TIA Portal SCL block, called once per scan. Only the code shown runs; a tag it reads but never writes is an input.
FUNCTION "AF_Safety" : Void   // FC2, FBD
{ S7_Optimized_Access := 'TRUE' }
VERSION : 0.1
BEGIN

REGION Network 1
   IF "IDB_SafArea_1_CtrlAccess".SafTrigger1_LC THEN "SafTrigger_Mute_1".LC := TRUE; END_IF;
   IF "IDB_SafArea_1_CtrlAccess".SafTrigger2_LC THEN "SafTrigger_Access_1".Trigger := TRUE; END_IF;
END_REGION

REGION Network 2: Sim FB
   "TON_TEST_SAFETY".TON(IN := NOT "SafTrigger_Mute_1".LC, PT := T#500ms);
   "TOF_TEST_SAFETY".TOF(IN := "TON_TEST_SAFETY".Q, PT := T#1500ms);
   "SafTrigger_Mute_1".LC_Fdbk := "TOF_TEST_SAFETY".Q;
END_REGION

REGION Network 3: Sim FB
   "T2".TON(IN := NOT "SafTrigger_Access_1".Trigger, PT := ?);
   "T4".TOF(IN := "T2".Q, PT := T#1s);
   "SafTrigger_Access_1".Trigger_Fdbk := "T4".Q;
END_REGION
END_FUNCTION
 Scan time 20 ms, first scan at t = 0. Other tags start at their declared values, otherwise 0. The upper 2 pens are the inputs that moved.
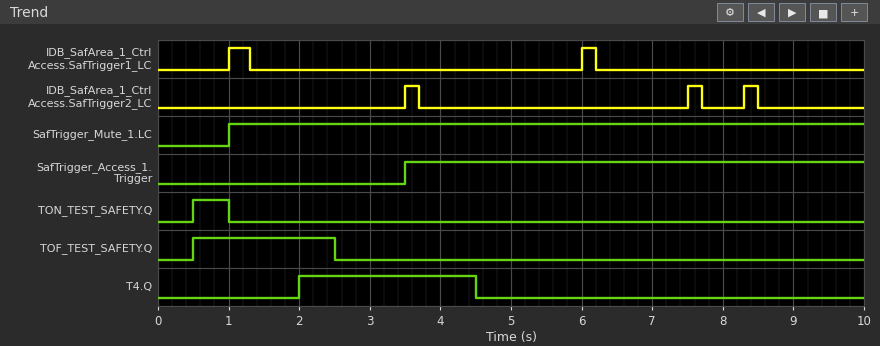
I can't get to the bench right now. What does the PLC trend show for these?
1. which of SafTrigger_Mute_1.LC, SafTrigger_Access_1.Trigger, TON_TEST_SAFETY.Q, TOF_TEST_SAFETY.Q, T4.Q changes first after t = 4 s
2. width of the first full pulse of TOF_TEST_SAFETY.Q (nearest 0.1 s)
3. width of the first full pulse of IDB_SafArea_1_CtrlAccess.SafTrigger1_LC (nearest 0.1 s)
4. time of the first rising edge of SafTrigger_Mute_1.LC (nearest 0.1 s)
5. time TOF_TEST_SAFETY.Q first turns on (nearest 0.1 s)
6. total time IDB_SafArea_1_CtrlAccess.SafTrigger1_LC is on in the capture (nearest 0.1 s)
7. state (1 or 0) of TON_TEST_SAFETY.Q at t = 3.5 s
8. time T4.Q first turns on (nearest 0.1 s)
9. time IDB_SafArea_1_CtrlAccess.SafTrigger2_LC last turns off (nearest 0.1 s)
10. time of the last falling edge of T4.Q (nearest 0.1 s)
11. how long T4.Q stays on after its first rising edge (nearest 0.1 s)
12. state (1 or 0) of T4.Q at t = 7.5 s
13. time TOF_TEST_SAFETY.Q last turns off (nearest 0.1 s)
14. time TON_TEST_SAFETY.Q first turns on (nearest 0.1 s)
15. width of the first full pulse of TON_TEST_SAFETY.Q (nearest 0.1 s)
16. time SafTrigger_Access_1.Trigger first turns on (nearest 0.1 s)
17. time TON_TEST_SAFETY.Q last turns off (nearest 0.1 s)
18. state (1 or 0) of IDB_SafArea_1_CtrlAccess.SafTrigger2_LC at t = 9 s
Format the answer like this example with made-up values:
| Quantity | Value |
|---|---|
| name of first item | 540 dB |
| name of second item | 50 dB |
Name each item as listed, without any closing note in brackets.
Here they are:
| Quantity | Value |
|---|---|
| which of SafTrigger_Mute_1.LC, SafTrigger_Access_1.Trigger, TON_TEST_SAFETY.Q, TOF_TEST_SAFETY.Q, T4.Q changes first after t = 4 s | T4.Q |
| width of the first full pulse of TOF_TEST_SAFETY.Q | 2.0 s |
| width of the first full pulse of IDB_SafArea_1_CtrlAccess.SafTrigger1_LC | 0.3 s |
| time of the first rising edge of SafTrigger_Mute_1.LC | 1.0 s |
| time TOF_TEST_SAFETY.Q first turns on | 0.5 s |
| total time IDB_SafArea_1_CtrlAccess.SafTrigger1_LC is on in the capture | 0.5 s |
| state (1 or 0) of TON_TEST_SAFETY.Q at t = 3.5 s | 0 |
| time T4.Q first turns on | 2.0 s |
| time IDB_SafArea_1_CtrlAccess.SafTrigger2_LC last turns off | 8.5 s |
| time of the last falling edge of T4.Q | 4.5 s |
| how long T4.Q stays on after its first rising edge | 2.5 s |
| state (1 or 0) of T4.Q at t = 7.5 s | 0 |
| time TOF_TEST_SAFETY.Q last turns off | 2.5 s |
| time TON_TEST_SAFETY.Q first turns on | 0.5 s |
| width of the first full pulse of TON_TEST_SAFETY.Q | 0.5 s |
| time SafTrigger_Access_1.Trigger first turns on | 3.5 s |
| time TON_TEST_SAFETY.Q last turns off | 1.0 s |
| state (1 or 0) of IDB_SafArea_1_CtrlAccess.SafTrigger2_LC at t = 9 s | 0 |
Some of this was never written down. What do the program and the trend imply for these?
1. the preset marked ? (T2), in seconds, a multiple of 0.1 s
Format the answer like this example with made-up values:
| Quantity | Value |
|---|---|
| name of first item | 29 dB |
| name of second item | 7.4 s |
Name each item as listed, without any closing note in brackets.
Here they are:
| Quantity | Value |
|---|---|
| the preset marked ? (T2), in seconds, a multiple of 0.1 s | 2.0 s |
